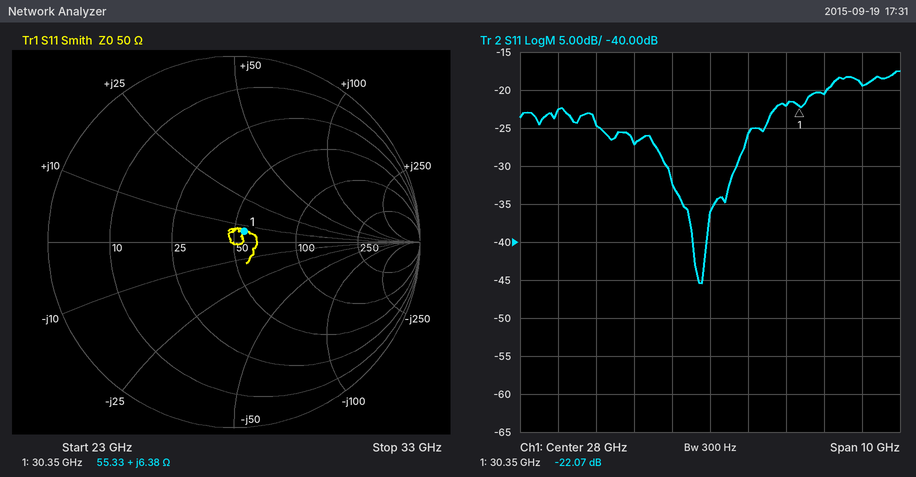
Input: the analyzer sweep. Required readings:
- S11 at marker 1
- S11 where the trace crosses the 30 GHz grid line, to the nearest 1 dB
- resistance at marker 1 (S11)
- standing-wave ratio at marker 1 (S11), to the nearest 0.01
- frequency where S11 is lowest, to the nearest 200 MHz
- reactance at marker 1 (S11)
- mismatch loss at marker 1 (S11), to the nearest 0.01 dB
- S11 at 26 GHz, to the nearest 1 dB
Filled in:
-22.07 dB
-22 dB
55.33 Ω
1.17
27.8 GHz
+6.38 Ω
0.03 dB
-27 dB
